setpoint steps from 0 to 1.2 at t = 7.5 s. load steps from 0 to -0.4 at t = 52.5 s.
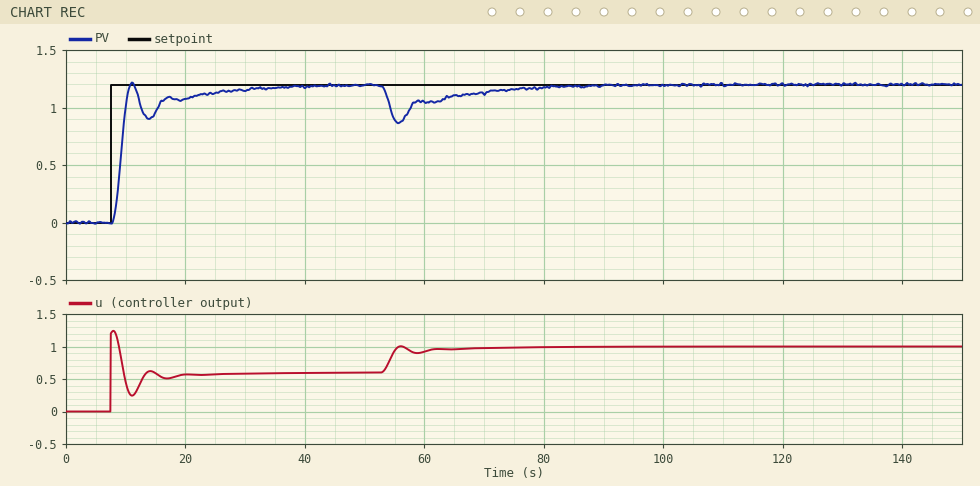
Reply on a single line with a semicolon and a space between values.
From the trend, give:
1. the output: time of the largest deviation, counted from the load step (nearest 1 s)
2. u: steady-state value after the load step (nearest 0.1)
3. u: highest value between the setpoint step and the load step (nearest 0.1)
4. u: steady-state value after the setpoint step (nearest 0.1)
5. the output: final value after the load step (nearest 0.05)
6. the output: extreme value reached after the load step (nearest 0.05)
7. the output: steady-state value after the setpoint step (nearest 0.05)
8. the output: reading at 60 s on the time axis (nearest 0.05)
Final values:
3 s; 1.0; 1.2; 0.6; 1.20; 0.85; 1.20; 1.05
